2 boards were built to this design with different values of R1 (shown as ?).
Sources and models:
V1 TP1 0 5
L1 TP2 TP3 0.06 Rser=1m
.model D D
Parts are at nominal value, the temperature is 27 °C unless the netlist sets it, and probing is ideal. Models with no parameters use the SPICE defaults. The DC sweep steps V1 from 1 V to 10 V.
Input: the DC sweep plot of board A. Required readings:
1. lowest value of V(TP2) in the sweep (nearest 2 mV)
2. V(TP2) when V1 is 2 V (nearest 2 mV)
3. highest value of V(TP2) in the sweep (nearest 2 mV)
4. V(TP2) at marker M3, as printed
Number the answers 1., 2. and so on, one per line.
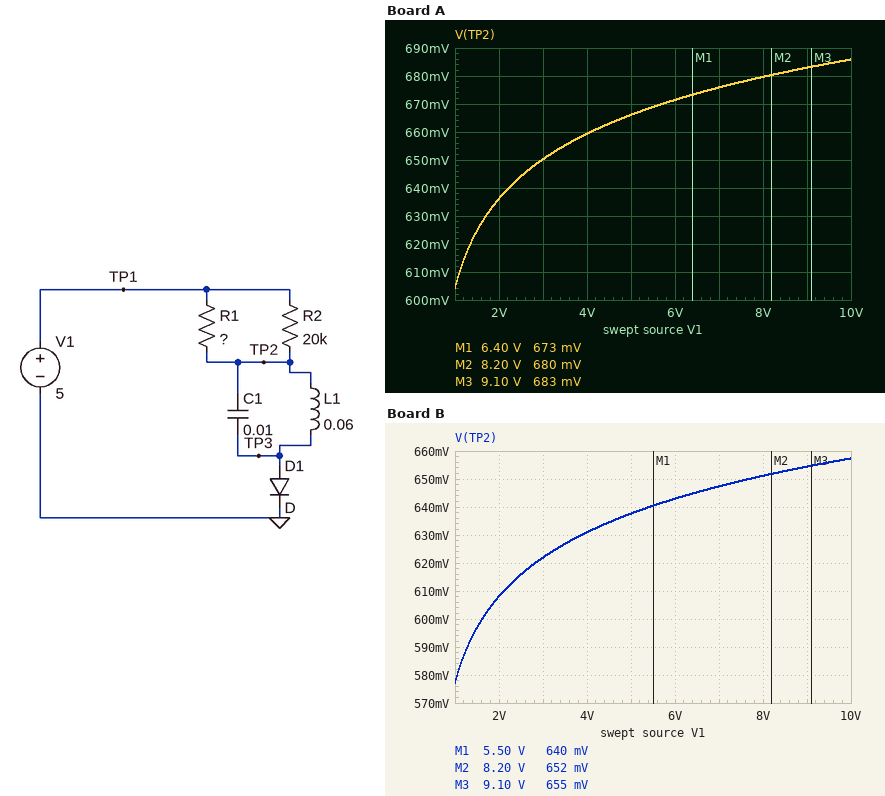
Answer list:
1. 604 mV
2. 636 mV
3. 686 mV
4. 683 mV
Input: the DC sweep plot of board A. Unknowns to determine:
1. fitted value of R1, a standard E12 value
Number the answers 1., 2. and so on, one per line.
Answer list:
1. 3.3 kΩ
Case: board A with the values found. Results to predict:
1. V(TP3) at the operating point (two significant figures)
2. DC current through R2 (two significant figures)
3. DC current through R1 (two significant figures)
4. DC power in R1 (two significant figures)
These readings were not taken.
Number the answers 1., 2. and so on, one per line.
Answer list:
1. 670 mV
2. 220 µA
3. 1.3 mA
4. 5.7 mW
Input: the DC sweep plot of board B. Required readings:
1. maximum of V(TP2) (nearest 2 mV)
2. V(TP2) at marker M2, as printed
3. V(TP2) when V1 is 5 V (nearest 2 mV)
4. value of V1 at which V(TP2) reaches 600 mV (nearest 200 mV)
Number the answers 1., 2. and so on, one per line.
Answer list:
1. 658 mV
2. 652 mV
3. 638 mV
4. 1.6 V
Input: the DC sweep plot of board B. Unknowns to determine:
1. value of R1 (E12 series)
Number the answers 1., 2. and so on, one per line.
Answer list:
1. 15 kΩ
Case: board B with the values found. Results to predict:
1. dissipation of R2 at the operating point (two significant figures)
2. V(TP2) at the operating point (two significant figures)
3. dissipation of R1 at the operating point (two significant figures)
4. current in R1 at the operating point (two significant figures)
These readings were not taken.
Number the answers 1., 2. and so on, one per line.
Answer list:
1. 950 µW
2. 640 mV
3. 1.3 mW
4. 290 µA
